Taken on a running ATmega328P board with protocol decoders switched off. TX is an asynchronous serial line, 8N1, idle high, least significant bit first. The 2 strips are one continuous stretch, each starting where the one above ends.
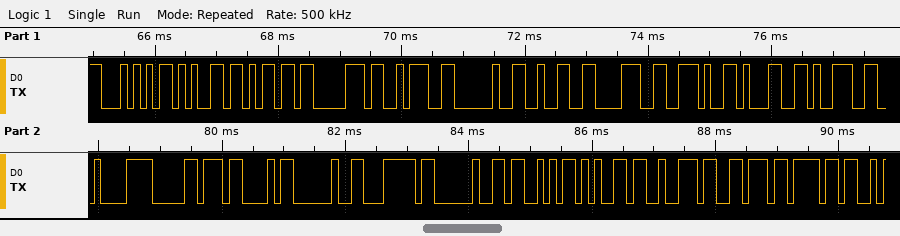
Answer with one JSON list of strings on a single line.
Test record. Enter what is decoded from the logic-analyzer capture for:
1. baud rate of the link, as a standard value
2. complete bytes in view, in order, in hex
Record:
["9600 baud", "54 65 6D 70 3A 20 32 38 2E 31 39 C2 B0 43 20 7C 20 53 65 72 76 6F"]
